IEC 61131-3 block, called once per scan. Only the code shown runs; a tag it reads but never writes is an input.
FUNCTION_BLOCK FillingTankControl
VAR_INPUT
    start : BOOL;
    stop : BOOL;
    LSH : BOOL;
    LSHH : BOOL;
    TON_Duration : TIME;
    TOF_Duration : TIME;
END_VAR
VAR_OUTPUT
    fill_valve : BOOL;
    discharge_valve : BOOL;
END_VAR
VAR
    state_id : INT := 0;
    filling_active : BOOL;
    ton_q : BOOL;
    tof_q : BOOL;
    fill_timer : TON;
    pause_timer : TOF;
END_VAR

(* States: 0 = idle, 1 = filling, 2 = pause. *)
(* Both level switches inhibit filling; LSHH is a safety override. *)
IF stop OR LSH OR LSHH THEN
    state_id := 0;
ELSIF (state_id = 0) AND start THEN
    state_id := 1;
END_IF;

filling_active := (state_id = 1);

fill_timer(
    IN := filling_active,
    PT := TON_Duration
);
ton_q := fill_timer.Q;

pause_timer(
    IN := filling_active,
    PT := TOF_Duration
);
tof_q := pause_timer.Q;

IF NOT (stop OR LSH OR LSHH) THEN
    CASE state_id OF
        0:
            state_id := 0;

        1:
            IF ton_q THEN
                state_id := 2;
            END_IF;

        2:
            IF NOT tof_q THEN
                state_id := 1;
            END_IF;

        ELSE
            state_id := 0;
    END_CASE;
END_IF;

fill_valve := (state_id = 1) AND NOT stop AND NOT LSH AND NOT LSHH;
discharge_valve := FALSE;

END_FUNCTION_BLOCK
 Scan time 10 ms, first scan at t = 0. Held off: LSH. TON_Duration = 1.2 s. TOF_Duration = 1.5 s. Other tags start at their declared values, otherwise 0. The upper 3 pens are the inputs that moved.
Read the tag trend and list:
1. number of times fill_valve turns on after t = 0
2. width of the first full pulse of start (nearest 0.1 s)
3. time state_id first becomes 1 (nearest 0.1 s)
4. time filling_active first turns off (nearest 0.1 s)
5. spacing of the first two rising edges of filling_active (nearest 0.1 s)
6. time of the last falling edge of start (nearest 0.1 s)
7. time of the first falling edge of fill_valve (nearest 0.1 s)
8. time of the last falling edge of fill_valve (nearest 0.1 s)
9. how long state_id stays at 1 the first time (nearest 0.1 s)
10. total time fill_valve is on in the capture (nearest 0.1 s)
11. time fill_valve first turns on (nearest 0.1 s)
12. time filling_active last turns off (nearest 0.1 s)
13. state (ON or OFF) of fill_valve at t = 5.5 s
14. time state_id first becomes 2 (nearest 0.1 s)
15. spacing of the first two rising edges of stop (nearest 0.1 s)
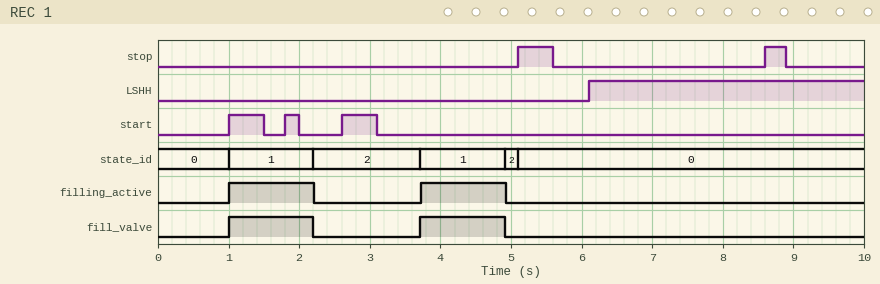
2
0.5 s
1.0 s
2.2 s
2.7 s
3.1 s
2.2 s
4.9 s
1.2 s
2.4 s
1.0 s
4.9 s
OFF
2.2 s
3.5 s
